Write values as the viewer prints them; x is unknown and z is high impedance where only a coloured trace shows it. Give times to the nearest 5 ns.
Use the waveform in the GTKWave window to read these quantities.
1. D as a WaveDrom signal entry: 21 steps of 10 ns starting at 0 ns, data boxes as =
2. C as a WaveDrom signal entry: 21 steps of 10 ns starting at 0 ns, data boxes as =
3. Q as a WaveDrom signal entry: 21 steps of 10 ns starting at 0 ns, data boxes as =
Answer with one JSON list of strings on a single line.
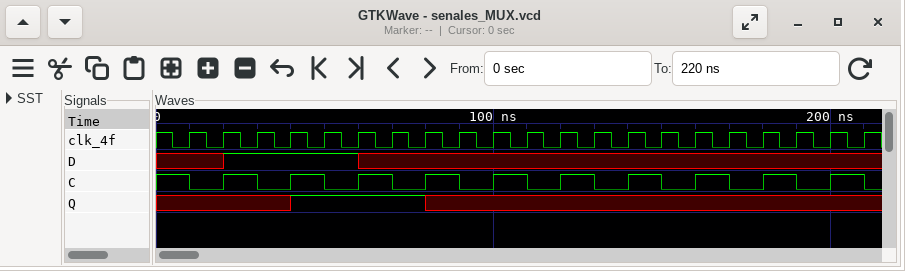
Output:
["{name: 'D', wave: 'x.1...x..............'}", "{name: 'C', wave: '101010101010101010101'}", "{name: 'Q', wave: 'x...1...x............'}"]
